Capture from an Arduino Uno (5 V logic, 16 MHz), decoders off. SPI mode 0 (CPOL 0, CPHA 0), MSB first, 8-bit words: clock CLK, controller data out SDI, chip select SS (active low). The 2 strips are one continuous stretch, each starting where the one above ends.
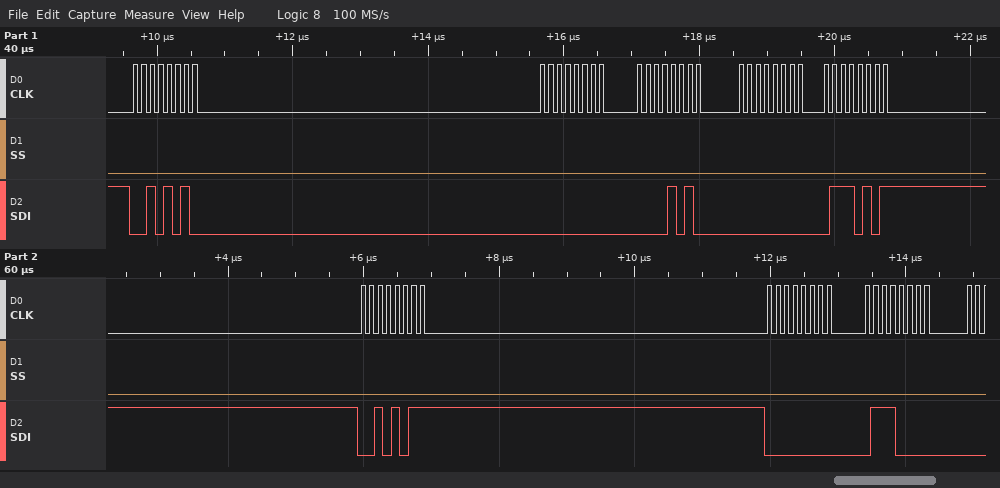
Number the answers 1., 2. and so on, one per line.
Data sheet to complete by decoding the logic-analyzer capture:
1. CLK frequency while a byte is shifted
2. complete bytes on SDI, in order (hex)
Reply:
1. 8 MHz
2. 2A 00 0A 00 75 2B 00 70
